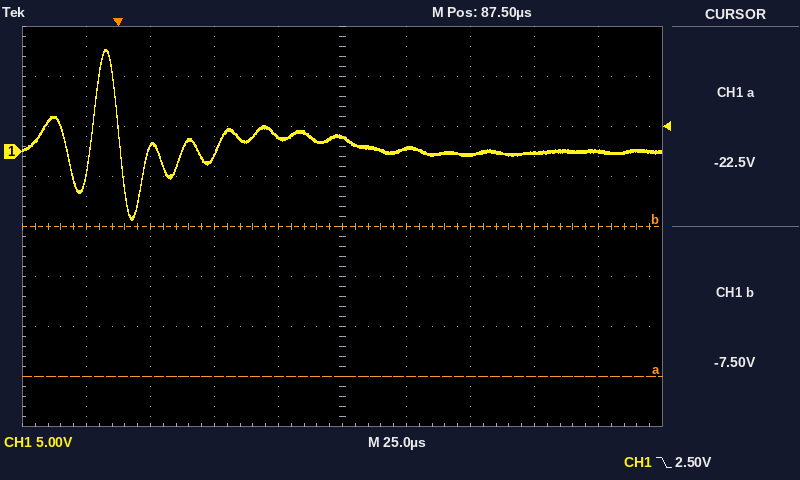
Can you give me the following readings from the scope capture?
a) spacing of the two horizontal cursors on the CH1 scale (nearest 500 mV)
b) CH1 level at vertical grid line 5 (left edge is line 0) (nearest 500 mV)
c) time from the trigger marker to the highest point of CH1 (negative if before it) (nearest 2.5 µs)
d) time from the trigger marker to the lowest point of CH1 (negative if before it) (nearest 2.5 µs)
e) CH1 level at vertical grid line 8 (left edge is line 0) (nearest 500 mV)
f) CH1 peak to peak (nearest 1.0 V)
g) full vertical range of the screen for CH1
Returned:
15.0 V
1.5 V
-5.0 µs
+5.0 µs
0.0 V
17.0 V
40 V
